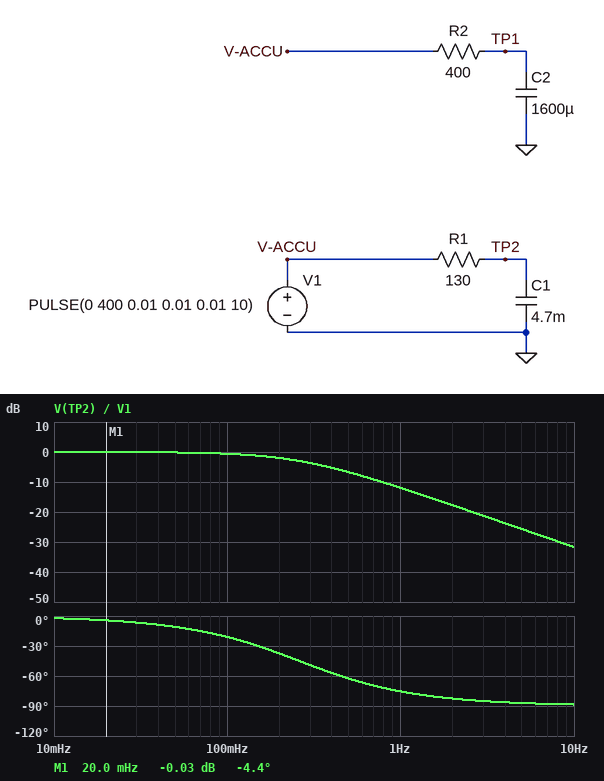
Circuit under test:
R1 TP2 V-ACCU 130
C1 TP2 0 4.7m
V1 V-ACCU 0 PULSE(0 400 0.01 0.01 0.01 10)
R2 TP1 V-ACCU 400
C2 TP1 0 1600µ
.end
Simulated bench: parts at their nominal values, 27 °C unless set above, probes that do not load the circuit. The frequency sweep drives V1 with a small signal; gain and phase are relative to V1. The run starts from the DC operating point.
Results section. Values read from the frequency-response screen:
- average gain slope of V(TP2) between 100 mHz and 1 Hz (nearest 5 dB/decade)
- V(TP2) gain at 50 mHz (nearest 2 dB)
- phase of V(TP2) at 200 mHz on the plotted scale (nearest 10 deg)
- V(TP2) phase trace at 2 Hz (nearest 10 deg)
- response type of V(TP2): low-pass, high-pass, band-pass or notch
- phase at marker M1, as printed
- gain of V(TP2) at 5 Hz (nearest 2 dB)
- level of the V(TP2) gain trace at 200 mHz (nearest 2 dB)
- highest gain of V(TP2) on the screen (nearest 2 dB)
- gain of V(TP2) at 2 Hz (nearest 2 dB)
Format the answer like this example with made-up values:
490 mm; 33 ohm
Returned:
-10 dB/decade; 0 dB; -40 deg; -80 deg; low-pass; -4.4 deg; -26 dB; -2 dB; 0 dB; -18 dB
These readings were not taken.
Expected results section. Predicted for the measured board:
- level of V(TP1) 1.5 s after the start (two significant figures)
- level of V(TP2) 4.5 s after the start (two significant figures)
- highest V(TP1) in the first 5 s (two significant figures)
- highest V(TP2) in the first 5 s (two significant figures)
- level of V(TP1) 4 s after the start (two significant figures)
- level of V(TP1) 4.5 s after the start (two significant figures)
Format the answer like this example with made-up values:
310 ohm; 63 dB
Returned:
360 V; 400 V; 400 V; 400 V; 400 V; 400 V
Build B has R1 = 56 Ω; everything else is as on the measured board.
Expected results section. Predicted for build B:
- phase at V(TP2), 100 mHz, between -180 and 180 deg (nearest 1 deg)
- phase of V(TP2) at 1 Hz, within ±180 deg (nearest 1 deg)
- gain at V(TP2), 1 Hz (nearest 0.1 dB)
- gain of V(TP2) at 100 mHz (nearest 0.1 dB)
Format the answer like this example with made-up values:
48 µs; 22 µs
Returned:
-9 deg; -59 deg; -5.7 dB; -0.1 dB
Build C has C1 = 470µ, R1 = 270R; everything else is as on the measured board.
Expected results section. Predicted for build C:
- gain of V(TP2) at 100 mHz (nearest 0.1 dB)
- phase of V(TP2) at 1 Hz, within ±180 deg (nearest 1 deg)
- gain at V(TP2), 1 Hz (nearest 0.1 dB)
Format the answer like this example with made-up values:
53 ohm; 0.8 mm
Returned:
0 dB; -39 deg; -2.1 dB
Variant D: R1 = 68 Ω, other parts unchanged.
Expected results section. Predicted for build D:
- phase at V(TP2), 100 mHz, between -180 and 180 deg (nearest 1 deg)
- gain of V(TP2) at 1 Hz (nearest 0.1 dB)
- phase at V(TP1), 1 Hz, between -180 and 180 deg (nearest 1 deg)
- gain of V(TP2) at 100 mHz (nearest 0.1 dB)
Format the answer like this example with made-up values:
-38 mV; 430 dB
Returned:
-11 deg; -7.0 dB; -76 deg; -0.2 dB
